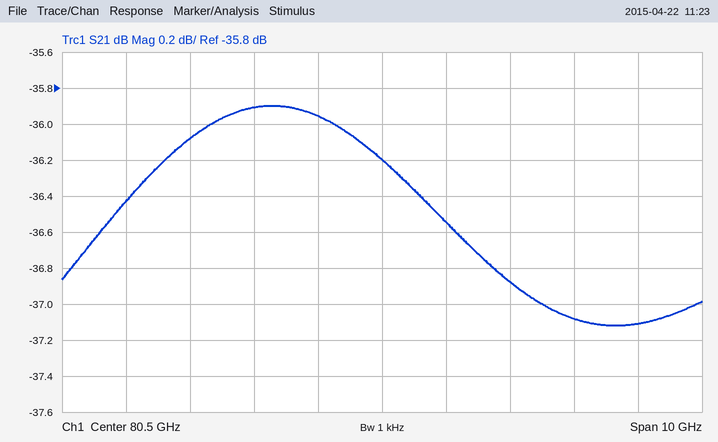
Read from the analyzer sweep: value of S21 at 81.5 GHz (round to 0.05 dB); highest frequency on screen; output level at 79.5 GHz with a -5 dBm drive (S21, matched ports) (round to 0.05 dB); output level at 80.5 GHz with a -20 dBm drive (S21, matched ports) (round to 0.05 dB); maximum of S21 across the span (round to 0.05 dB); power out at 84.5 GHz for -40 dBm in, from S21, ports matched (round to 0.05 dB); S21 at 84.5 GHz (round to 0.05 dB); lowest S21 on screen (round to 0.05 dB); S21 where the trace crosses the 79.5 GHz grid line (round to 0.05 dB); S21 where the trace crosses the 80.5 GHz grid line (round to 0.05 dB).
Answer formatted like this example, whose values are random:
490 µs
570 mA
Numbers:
-36.55 dB
85.5 GHz
-40.95 dBm
-56.20 dBm
-35.90 dB
-77.10 dBm
-37.10 dB
-37.10 dB
-35.95 dB
-36.20 dB
